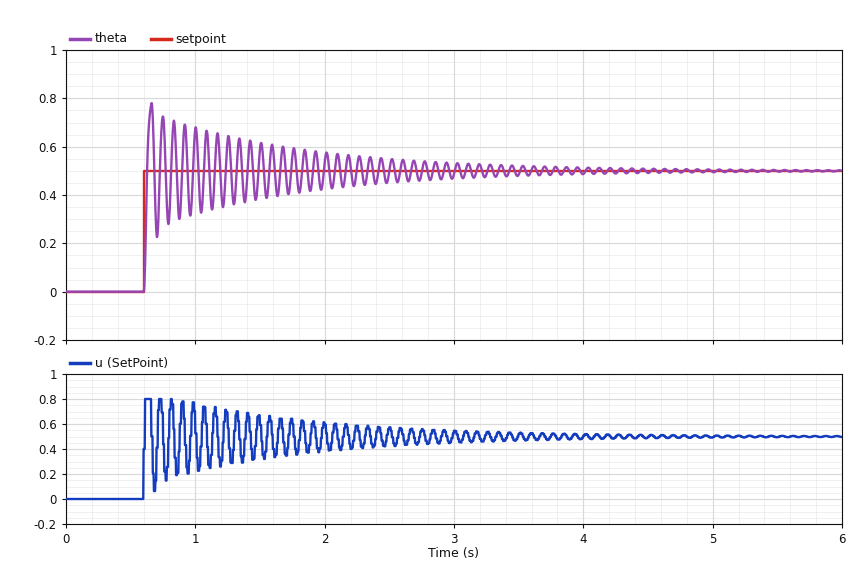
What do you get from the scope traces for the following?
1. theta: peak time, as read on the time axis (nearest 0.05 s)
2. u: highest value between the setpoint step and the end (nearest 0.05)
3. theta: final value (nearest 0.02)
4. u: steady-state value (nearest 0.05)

0.65 s
0.80
0.50
0.50
